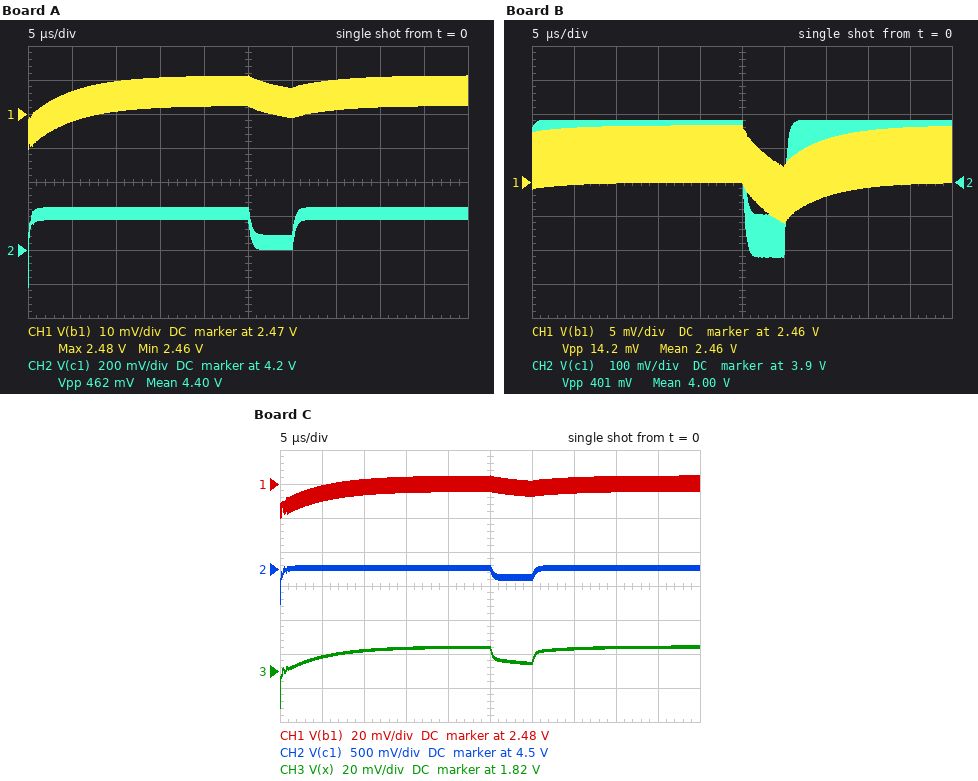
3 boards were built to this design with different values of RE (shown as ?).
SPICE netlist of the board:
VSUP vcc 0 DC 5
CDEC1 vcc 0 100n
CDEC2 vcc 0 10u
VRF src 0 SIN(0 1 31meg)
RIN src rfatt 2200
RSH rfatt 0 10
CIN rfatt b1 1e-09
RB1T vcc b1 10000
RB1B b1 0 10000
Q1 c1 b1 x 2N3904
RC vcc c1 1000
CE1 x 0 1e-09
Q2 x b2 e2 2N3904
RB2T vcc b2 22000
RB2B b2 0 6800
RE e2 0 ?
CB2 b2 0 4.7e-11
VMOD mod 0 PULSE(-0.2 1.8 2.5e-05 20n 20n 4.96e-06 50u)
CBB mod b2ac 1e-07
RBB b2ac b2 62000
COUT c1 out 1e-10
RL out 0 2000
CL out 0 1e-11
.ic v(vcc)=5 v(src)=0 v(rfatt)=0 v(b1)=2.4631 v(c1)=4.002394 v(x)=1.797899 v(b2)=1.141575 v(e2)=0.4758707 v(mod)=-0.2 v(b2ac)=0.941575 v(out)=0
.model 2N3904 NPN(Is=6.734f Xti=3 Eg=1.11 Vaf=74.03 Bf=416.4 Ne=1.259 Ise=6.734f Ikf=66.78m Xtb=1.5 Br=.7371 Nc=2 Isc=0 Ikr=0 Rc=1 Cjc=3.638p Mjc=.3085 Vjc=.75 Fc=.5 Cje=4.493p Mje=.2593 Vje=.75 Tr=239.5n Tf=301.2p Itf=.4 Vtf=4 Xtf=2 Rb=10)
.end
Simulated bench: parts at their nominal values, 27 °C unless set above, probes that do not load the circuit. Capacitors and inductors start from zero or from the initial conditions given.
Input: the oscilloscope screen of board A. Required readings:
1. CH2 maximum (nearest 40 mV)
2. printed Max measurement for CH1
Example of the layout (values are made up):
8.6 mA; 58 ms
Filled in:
4.44 V; 2.48 V
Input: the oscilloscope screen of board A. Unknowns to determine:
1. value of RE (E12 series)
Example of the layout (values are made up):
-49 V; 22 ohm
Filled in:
820 Ω
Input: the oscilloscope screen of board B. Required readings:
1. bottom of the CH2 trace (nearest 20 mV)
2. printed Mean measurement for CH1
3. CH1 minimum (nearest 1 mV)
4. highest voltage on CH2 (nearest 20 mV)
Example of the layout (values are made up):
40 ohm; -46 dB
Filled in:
3.68 V; 2.46 V; 2.454 V; 4.08 V
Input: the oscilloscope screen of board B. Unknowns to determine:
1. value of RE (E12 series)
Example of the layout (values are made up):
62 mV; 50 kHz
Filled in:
470 Ω
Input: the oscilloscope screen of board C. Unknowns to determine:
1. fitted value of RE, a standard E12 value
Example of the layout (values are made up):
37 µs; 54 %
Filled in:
1 kΩ
